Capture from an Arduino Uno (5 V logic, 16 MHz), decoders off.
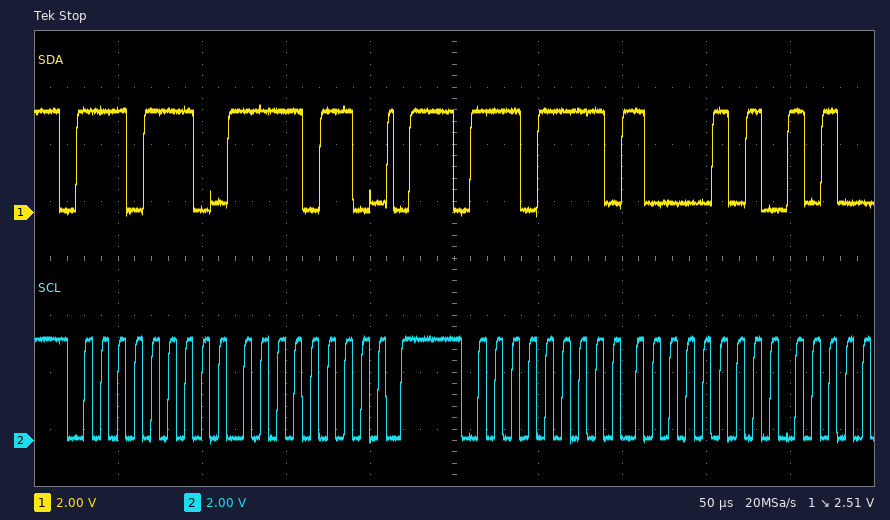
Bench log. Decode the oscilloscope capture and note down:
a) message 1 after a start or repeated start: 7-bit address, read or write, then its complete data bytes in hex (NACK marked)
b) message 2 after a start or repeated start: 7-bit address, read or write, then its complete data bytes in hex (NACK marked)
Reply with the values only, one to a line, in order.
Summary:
0x77 write: F6
0x77 read: 85
